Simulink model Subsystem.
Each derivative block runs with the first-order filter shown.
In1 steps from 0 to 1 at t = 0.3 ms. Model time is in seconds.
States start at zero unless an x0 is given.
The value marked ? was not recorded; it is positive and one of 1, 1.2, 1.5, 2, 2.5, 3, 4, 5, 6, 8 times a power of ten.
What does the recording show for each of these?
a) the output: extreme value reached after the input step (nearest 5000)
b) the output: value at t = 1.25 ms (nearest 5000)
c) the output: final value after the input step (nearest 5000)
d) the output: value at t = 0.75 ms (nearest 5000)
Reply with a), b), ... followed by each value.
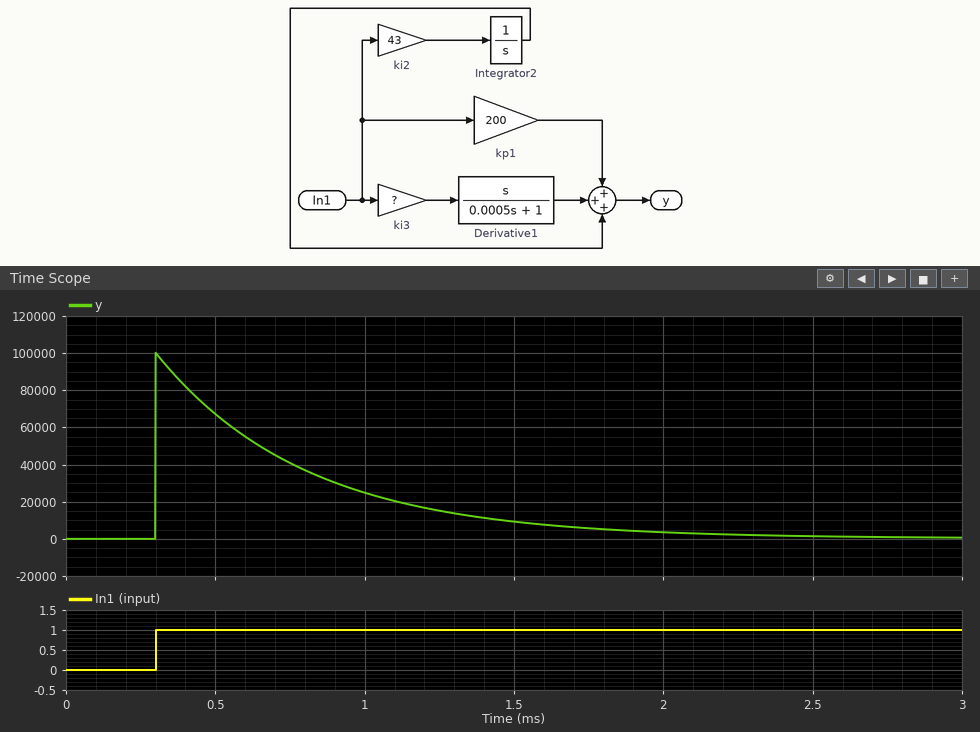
a) 100000
b) 15000
c) 0
d) 40000
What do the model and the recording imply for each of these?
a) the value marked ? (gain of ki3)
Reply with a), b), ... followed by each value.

a) 50
